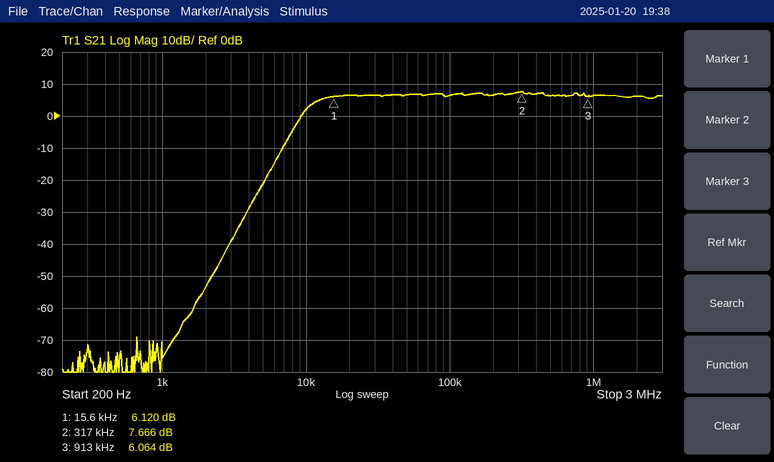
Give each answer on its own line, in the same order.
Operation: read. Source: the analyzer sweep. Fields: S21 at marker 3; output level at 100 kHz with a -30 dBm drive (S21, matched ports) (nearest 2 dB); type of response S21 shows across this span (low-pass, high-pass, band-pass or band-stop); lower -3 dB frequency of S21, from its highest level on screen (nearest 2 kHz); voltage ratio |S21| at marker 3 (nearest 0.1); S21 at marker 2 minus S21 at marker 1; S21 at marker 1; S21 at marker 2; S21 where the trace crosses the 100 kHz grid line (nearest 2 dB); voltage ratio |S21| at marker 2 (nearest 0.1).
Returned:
6.064 dB
-24 dBm
high-pass
12 kHz
2.0
1.546 dB
6.120 dB
7.666 dB
6 dB
2.4
